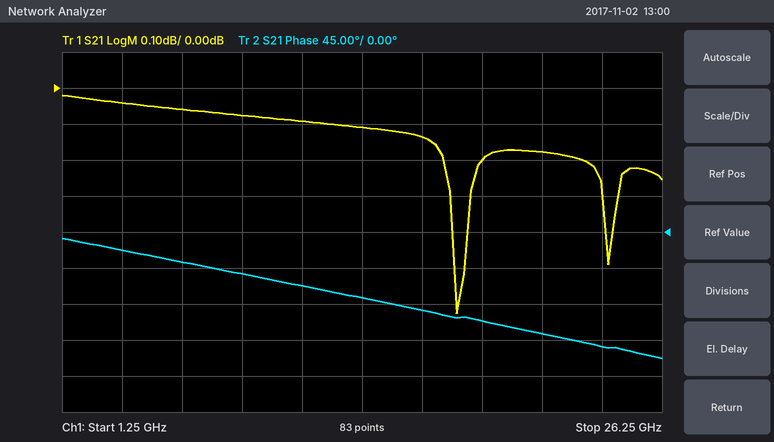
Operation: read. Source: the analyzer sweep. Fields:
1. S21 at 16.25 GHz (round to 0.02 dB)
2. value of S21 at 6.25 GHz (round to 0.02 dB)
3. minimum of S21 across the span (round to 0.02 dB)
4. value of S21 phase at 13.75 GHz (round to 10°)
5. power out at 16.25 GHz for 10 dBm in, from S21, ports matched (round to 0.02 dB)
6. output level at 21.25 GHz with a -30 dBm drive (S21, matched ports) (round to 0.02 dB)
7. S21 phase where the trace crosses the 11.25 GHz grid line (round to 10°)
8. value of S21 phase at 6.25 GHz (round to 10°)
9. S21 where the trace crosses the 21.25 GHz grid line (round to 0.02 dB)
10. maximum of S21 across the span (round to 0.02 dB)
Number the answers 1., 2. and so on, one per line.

1. -0.14 dB
2. -0.06 dB
3. -0.62 dB
4. -80°
5. 9.86 dBm
6. -30.18 dBm
7. -70°
8. -40°
9. -0.18 dB
10. -0.02 dB
